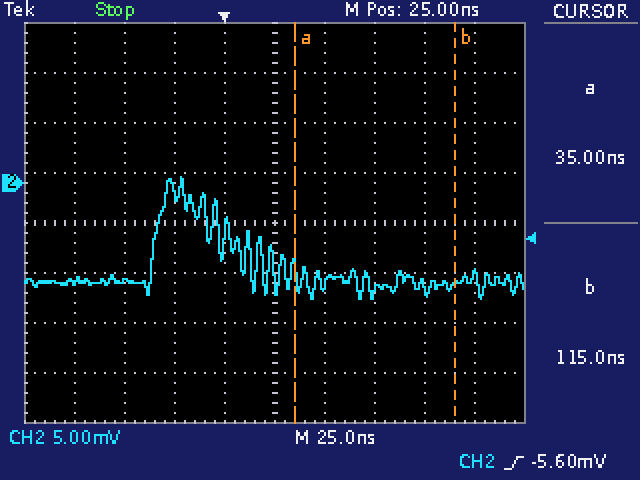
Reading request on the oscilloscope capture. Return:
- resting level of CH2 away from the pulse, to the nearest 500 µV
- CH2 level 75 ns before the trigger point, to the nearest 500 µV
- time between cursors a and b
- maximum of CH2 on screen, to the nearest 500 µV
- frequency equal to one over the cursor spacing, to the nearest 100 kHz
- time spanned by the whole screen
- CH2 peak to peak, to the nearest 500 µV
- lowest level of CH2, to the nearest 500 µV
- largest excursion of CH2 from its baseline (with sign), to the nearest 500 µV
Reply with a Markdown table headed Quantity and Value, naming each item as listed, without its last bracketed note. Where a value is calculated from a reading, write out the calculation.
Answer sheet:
| Quantity | Value |
|---|---|
| resting level of CH2 away from the pulse, to the nearest 500 µV | -10.0 mV |
| CH2 level 75 ns before the trigger point, to the nearest 500 µV | -10.0 mV |
| time between cursors a and b | 115 ns − (35 ns) = 80.0 ns |
| maximum of CH2 on screen, to the nearest 500 µV | 500 µV |
| frequency equal to one over the cursor spacing, to the nearest 100 kHz | 1 / 80.0 ns ≈ 12.5 MHz |
| time spanned by the whole screen | 250 ns |
| CH2 peak to peak, to the nearest 500 µV | 500 µV − (-11.5 mV) = 12.0 mV |
| lowest level of CH2, to the nearest 500 µV | -11.5 mV |
| largest excursion of CH2 from its baseline (with sign), to the nearest 500 µV | 500 µV − (-10.0 mV) = +10.5 mV |
